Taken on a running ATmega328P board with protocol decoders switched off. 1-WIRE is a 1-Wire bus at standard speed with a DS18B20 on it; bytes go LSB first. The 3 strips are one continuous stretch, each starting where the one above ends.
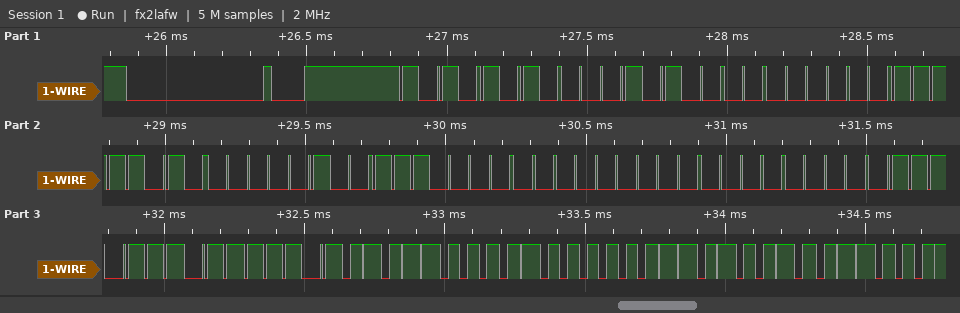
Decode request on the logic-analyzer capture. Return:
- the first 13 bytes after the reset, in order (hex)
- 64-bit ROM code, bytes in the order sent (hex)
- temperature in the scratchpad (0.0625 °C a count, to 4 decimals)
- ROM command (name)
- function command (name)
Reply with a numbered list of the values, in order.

1. 55 28 00 5F 20 07 00 00 EE BE 1A 02 4B
2. 28 00 5F 20 07 00 00 EE
3. 33.6250 °C
4. Match ROM
5. Read Scratchpad
